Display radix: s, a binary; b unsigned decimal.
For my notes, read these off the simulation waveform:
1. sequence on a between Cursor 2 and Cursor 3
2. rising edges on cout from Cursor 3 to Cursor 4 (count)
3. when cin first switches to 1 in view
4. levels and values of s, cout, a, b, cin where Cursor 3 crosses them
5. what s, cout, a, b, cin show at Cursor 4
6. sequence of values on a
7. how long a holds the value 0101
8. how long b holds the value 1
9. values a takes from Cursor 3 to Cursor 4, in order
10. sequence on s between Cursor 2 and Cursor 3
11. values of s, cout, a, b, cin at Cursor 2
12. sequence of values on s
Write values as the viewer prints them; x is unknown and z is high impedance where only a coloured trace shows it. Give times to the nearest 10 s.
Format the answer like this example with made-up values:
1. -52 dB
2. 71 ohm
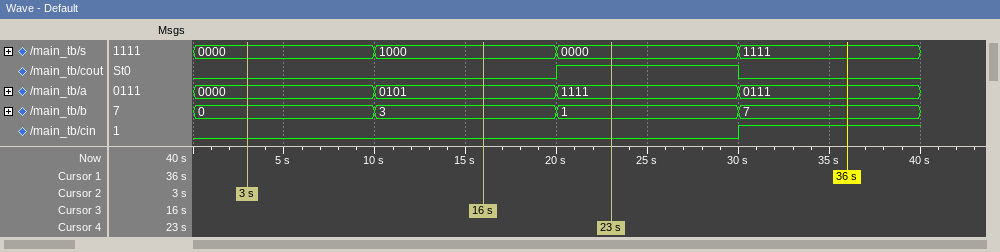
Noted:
1. 0000, 0101
2. 1
3. 30 s
4. s=1000, cout=0, a=0101, b=3, cin=0
5. s=0000, cout=1, a=1111, b=1, cin=0
6. 0000, 0101, 1111, 0111
7. 10 s
8. 10 s
9. 0101, 1111
10. 0000, 1000
11. s=0000, cout=0, a=0000, b=0, cin=0
12. 0000, 1000, 0000, 1111
